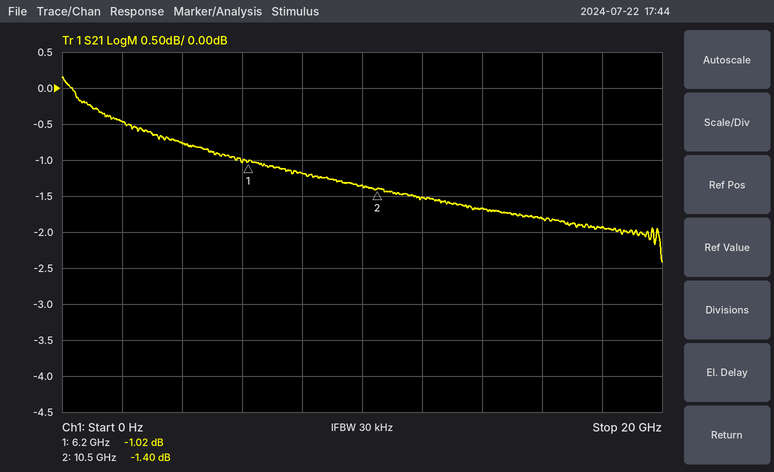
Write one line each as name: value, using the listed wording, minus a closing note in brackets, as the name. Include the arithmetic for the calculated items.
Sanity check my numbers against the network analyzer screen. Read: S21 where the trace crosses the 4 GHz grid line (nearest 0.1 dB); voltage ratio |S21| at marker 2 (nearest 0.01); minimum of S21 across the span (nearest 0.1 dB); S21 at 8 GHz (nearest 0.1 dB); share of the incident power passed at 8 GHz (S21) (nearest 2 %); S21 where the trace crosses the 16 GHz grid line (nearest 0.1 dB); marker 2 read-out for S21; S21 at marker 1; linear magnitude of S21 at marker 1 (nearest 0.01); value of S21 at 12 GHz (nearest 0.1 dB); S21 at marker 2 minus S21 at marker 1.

S21 where the trace crosses the 4 GHz grid line: -0.8 dB
voltage ratio |S21| at marker 2: 10^(-1.4/20) ≈ 0.85
minimum of S21 across the span: -2.4 dB
S21 at 8 GHz: -1.2 dB
share of the incident power passed at 8 GHz (S21): 10^(-1.2/10) ≈ 76 %
S21 where the trace crosses the 16 GHz grid line: -1.8 dB
marker 2 read-out for S21: -1.40 dB
S21 at marker 1: -1.02 dB
linear magnitude of S21 at marker 1: 10^(-1.02/20) ≈ 0.89
value of S21 at 12 GHz: -1.5 dB
S21 at marker 2 minus S21 at marker 1: -1.4 − (-1.02) = -0.38 dB
